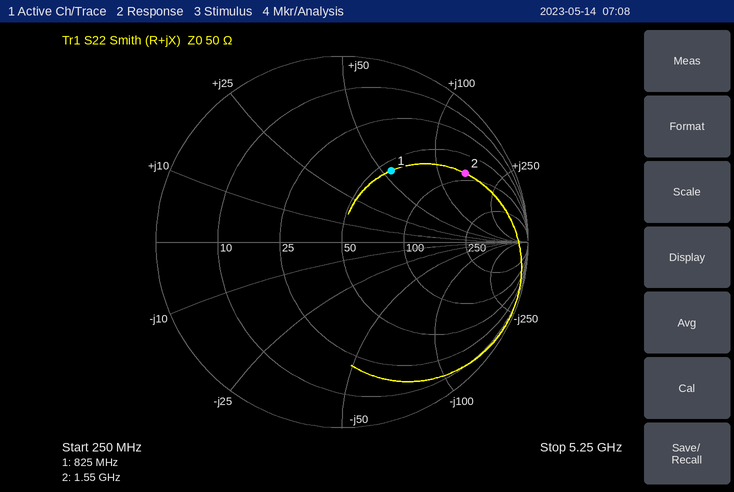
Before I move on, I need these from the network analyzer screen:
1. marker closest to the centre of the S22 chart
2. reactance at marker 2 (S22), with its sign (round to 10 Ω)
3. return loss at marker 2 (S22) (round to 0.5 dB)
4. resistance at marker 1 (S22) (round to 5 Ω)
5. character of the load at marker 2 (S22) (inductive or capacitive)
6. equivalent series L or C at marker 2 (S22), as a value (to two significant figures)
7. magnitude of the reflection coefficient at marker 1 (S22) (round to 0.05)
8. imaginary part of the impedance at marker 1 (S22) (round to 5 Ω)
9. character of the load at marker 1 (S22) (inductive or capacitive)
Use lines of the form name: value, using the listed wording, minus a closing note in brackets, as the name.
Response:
marker closest to the centre of the S22 chart: marker 1
reactance at marker 2 (S22), with its sign: +150 Ω
return loss at marker 2 (S22): 2.5 dB
resistance at marker 1 (S22): 55 Ω
character of the load at marker 2 (S22): inductive
equivalent series L or C at marker 2 (S22), as a value: 15 nH
magnitude of the reflection coefficient at marker 1 (S22): 0.45
imaginary part of the impedance at marker 1 (S22): +55 Ω
character of the load at marker 1 (S22): inductive
